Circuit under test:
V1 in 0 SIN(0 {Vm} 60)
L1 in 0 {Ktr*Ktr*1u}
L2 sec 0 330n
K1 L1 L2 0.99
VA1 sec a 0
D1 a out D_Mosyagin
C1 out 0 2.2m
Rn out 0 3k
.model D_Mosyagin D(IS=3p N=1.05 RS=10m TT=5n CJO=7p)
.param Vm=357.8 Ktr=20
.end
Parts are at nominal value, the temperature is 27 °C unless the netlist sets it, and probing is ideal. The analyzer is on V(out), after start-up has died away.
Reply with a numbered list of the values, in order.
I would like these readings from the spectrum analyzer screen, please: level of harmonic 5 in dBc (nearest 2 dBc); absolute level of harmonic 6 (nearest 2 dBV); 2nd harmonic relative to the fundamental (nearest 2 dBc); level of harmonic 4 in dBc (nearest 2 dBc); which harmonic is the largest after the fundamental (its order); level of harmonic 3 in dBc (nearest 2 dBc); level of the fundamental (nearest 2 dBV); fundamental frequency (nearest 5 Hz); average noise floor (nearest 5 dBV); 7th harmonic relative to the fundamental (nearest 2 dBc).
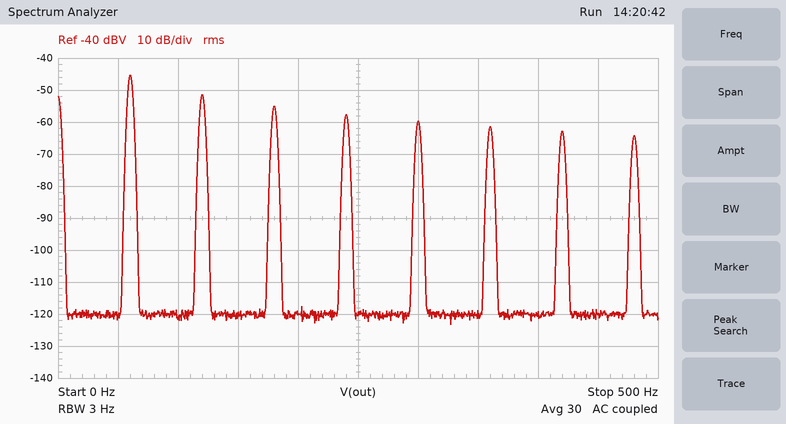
1. -14 dBc
2. -62 dBV
3. -6 dBc
4. -12 dBc
5. 2
6. -10 dBc
7. -46 dBV
8. 60 Hz
9. -120 dBV
10. -18 dBc
